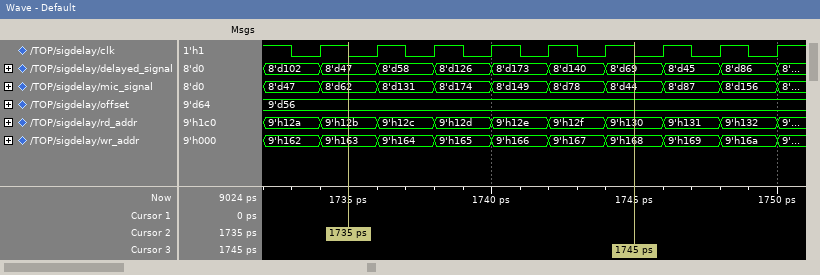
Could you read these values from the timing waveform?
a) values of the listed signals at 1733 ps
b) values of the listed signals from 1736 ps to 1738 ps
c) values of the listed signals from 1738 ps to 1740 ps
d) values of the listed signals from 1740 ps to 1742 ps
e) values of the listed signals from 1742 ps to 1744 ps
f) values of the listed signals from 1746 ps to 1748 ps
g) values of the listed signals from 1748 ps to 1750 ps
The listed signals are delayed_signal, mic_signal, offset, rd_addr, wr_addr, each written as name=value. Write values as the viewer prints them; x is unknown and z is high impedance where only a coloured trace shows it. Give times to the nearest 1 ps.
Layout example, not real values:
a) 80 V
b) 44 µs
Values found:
a) delayed_signal=8'd102, mic_signal=8'd47, offset=9'd56, rd_addr=9'h12a, wr_addr=9'h162
b) delayed_signal=8'd58, mic_signal=8'd131, offset=9'd56, rd_addr=9'h12c, wr_addr=9'h164
c) delayed_signal=8'd126, mic_signal=8'd174, offset=9'd56, rd_addr=9'h12d, wr_addr=9'h165
d) delayed_signal=8'd173, mic_signal=8'd149, offset=9'd56, rd_addr=9'h12e, wr_addr=9'h166
e) delayed_signal=8'd140, mic_signal=8'd78, offset=9'd56, rd_addr=9'h12f, wr_addr=9'h167
f) delayed_signal=8'd45, mic_signal=8'd87, offset=9'd56, rd_addr=9'h131, wr_addr=9'h169
g) delayed_signal=8'd86, mic_signal=8'd156, offset=9'd56, rd_addr=9'h132, wr_addr=9'h16a
